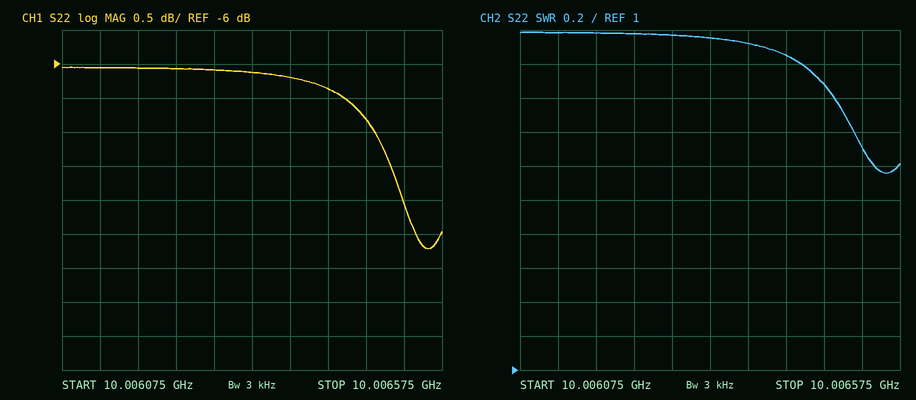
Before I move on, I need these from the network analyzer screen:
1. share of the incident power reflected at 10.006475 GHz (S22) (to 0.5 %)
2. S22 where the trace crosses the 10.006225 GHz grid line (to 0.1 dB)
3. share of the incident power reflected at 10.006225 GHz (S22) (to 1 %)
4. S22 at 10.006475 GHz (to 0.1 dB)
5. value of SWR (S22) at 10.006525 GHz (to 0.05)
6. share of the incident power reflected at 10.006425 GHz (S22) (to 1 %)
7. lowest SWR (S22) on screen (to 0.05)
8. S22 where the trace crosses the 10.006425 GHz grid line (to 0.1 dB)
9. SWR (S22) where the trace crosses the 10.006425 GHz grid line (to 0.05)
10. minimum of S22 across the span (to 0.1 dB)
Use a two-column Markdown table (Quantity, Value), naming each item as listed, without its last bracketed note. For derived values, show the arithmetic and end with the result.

| Quantity | Value |
|---|---|
| share of the incident power reflected at 10.006475 GHz (S22) | 10^(-6.8/10) ≈ 20.9 %, so 21.0 % to the nearest 0.5 % |
| S22 where the trace crosses the 10.006225 GHz grid line | -6.1 dB |
| share of the incident power reflected at 10.006225 GHz (S22) | 10^(-6.1/10) ≈ 25 % |
| S22 at 10.006475 GHz | -6.8 dB |
| value of SWR (S22) at 10.006525 GHz | 2.30 |
| share of the incident power reflected at 10.006425 GHz (S22) | 10^(-6.4/10) ≈ 23 % |
| lowest SWR (S22) on screen | 2.15 |
| S22 where the trace crosses the 10.006425 GHz grid line | -6.4 dB |
| SWR (S22) where the trace crosses the 10.006425 GHz grid line | 2.85 |
| minimum of S22 across the span | -8.7 dB |
